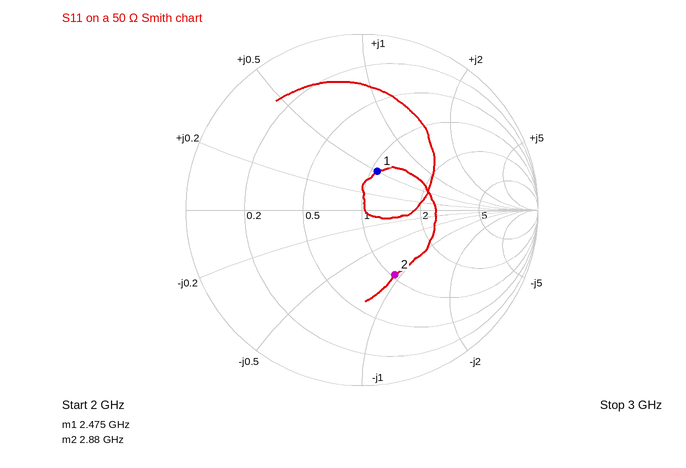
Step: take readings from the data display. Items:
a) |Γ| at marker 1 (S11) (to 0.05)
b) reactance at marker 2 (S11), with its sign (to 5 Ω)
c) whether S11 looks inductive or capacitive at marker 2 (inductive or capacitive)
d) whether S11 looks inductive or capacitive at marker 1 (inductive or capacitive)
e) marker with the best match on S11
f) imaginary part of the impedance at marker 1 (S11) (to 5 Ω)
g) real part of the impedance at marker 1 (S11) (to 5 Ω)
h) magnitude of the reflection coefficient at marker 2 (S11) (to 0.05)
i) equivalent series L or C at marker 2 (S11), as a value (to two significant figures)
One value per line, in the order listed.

0.25
-45 Ω
capacitive
inductive
marker 1
+25 Ω
55 Ω
0.40
1.2 pF
